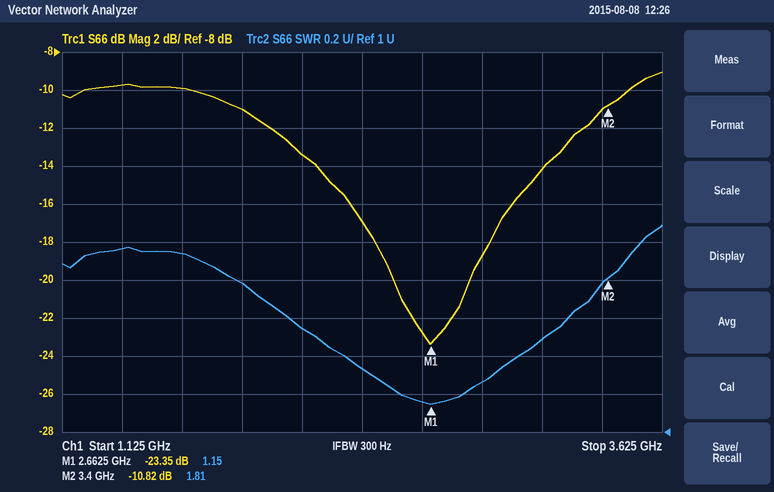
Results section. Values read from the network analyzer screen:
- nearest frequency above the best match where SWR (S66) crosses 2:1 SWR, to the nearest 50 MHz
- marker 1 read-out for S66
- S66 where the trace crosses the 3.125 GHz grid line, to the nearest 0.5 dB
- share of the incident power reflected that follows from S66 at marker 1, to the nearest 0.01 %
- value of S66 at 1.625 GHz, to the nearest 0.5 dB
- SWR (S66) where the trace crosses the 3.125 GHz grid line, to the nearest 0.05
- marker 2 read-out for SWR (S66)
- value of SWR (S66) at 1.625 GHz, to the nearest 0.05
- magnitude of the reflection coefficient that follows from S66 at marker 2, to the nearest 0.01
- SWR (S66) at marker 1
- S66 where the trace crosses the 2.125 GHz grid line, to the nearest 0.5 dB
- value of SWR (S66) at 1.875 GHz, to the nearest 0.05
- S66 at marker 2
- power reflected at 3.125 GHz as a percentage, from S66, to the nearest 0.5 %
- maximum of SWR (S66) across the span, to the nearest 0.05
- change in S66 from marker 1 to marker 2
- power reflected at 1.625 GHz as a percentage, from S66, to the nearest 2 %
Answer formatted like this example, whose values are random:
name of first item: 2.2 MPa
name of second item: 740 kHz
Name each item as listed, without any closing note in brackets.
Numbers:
nearest frequency above the best match where SWR (S66) crosses 2:1 SWR, to the nearest 50 MHz: 3.55 GHz
marker 1 read-out for S66: -23.35 dB
S66 where the trace crosses the 3.125 GHz grid line, to the nearest 0.5 dB: -14.0 dB
share of the incident power reflected that follows from S66 at marker 1, to the nearest 0.01 %: 0.46 %
value of S66 at 1.625 GHz, to the nearest 0.5 dB: -10.0 dB
SWR (S66) where the trace crosses the 3.125 GHz grid line, to the nearest 0.05: 1.50
marker 2 read-out for SWR: 1.81
value of SWR (S66) at 1.625 GHz, to the nearest 0.05: 1.95
magnitude of the reflection coefficient that follows from S66 at marker 2, to the nearest 0.01: 0.29
SWR (S66) at marker 1: 1.15
S66 where the trace crosses the 2.125 GHz grid line, to the nearest 0.5 dB: -13.5 dB
value of SWR (S66) at 1.875 GHz, to the nearest 0.05: 1.80
S66 at marker 2: -10.82 dB
power reflected at 3.125 GHz as a percentage, from S66, to the nearest 0.5 %: 4.0 %
maximum of SWR (S66) across the span, to the nearest 0.05: 2.10
change in S66 from marker 1 to marker 2: 12.53 dB
power reflected at 1.625 GHz as a percentage, from S66, to the nearest 2 %: 10 %
